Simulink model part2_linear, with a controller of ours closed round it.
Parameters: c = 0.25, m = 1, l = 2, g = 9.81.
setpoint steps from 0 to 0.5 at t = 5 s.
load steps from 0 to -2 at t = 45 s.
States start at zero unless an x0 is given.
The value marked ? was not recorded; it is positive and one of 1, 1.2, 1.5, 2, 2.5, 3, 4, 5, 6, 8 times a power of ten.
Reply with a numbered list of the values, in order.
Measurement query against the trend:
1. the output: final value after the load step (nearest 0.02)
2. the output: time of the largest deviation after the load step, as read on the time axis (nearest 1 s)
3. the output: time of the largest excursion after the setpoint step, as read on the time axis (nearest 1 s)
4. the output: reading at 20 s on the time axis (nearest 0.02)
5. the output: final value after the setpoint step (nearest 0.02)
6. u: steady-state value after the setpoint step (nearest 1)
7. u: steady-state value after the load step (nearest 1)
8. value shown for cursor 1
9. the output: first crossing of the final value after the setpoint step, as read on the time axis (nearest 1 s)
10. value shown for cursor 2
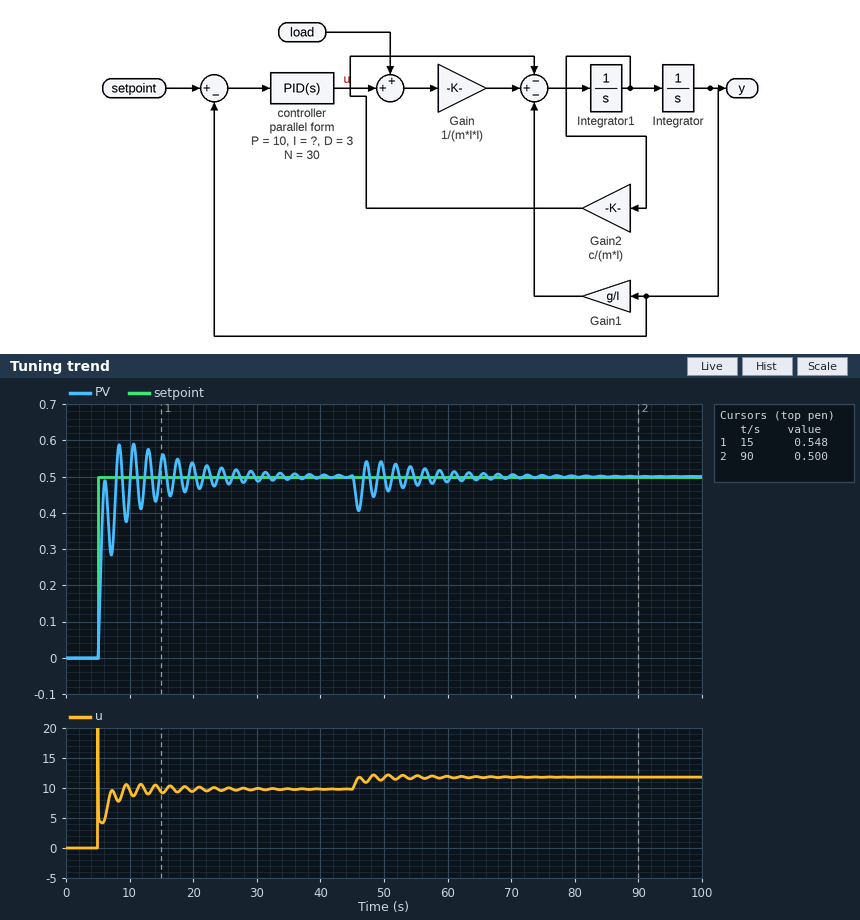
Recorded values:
1. 0.50
2. 46 s
3. 11 s
4. 0.54
5. 0.50
6. 10
7. 12
8. 0.548
9. 8 s
10. 0.500
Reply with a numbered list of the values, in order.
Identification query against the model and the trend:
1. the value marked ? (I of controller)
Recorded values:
1. 20
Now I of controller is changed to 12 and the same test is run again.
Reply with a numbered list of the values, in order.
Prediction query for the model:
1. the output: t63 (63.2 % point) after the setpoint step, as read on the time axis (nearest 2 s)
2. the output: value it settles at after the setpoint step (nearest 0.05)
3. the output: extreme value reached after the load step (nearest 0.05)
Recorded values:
1. 6 s
2. 0.50
3. 0.40
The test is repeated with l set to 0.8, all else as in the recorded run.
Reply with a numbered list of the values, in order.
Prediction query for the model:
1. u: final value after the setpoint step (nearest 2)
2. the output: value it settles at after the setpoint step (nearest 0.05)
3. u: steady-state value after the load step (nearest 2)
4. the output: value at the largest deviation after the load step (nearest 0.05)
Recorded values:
1. 4
2. 0.50
3. 6
4. 0.40
